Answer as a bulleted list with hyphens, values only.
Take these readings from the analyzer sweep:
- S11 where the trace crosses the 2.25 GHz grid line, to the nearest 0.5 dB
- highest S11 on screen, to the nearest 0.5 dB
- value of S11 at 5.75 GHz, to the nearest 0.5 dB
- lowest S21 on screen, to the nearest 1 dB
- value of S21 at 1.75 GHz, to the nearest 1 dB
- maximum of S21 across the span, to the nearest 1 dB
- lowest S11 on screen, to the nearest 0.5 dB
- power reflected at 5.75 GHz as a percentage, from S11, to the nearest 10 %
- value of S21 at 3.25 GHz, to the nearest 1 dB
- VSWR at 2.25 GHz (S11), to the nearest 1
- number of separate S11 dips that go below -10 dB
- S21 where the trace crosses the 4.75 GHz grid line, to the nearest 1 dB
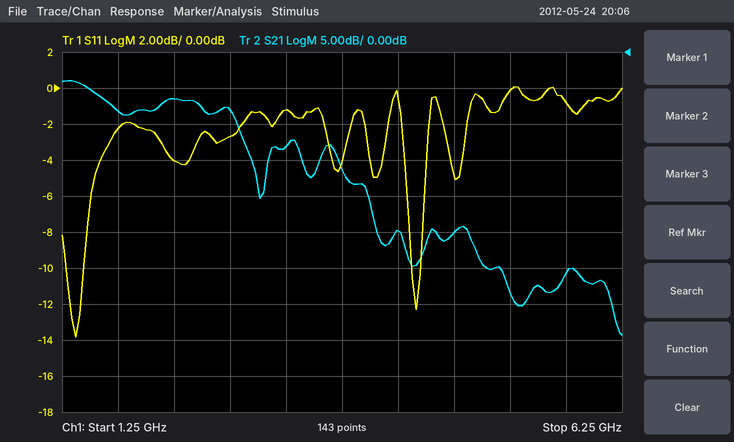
- -4.0 dB
- 0.0 dB
- -1.0 dB
- -39 dB
- -8 dB
- -4 dB
- -14.0 dB
- 80 %
- -13 dB
- 4
- 2
- -25 dB
